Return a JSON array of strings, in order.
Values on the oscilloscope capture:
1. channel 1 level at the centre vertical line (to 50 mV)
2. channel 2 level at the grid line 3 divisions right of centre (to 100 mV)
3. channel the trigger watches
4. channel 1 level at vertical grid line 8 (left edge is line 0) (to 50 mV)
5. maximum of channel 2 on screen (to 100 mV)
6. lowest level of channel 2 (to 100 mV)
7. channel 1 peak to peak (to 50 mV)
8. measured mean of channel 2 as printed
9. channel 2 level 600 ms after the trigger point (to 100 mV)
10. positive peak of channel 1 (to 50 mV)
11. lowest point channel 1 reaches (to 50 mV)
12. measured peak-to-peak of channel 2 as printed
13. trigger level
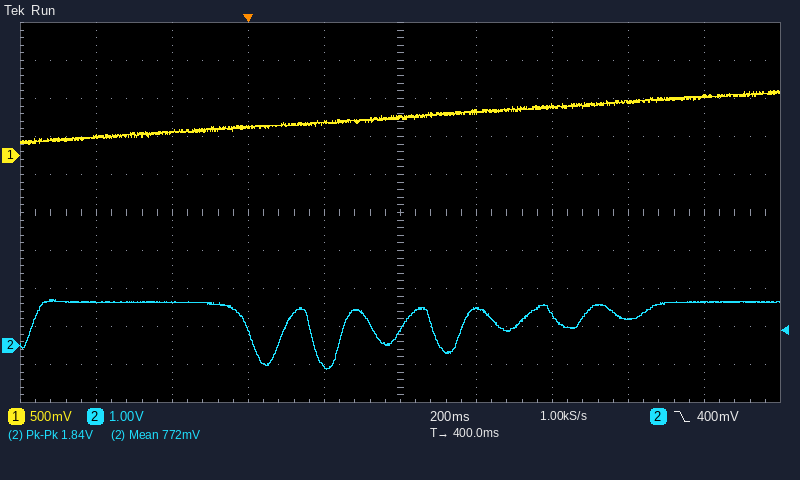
["500 mV", "700 mV", "channel 2", "700 mV", "1.2 V", "-600 mV", "700 mV", "772 mV", "1.0 V", "850 mV", "150 mV", "1.84 V", "400 mV"]
